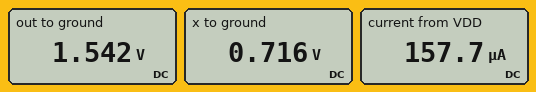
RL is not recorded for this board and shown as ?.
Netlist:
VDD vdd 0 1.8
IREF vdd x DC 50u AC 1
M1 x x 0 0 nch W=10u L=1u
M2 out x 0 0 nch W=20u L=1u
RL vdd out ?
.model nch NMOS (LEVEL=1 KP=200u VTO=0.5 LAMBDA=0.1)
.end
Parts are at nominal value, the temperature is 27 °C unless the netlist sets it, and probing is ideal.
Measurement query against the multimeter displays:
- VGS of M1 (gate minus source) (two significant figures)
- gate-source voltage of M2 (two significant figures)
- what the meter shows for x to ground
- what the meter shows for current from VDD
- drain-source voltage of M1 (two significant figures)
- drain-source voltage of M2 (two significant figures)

720 mV
720 mV
0.716 V
157.7 µA
720 mV
1.5 V
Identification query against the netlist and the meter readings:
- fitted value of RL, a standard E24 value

2.4 kΩ
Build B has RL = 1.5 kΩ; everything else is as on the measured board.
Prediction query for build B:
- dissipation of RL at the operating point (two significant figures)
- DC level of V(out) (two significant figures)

18 µW
1.6 V
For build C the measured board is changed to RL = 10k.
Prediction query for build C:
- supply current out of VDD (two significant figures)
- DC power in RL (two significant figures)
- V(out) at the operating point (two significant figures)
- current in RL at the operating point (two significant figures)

150 µA
100 µW
790 mV
100 µA
